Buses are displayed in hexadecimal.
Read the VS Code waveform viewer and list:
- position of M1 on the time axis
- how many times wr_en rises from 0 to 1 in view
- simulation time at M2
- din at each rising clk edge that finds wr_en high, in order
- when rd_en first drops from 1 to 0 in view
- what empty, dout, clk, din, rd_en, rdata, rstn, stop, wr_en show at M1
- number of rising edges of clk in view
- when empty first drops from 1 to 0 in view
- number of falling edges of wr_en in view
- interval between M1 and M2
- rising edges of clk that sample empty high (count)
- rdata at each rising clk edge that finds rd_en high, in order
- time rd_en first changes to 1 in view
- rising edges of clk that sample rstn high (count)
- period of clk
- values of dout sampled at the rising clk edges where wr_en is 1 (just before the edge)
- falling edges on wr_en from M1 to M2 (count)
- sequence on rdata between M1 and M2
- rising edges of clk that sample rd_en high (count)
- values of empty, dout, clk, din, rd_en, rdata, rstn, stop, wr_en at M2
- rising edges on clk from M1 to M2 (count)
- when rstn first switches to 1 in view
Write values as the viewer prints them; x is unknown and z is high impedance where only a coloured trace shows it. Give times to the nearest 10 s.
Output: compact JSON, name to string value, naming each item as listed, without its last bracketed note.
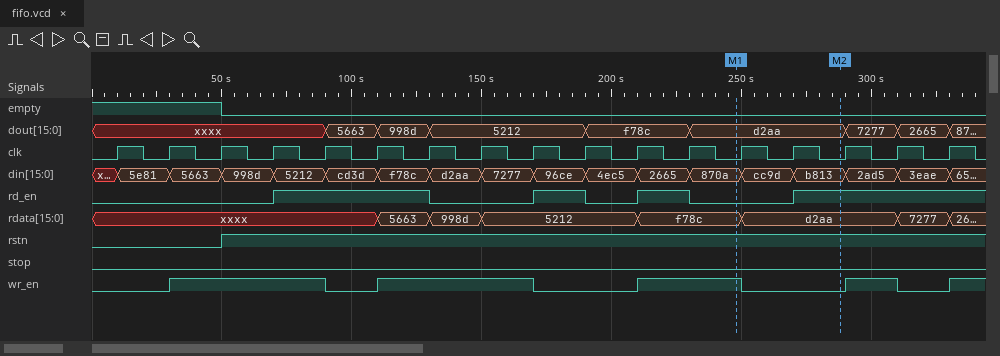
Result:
{"position of M1 on the time axis": "250 s", "how many times wr_en rises from 0 to 1 in view": "5", "simulation time at M2": "290 s", "din at each rising clk edge that finds wr_en high, in order": "5663, 998d, 5212, f78c, d2aa, 7277, 2665, 870a, 2ad5", "when rd_en first drops from 1 to 0 in view": "130 s", "what empty, dout, clk, din, rd_en, rdata, rstn, stop, wr_en show at M1": "empty=0, dout=d2aa, clk=0, din=870a, rd_en=0, rdata=f78c, rstn=1, stop=0, wr_en=1", "number of rising edges of clk in view": "17", "when empty first drops from 1 to 0 in view": "50 s", "number of falling edges of wr_en in view": "4", "interval between M1 and M2": "40 s", "rising edges of clk that sample empty high": "3", "rdata at each rising clk edge that finds rd_en high, in order": "xxxx, xxxx, 5663, 5212, f78c, d2aa, d2aa, 7277", "time rd_en first changes to 1 in view": "70 s", "rising edges of clk that sample rstn high": "14", "period of clk": "20 s", "values of dout sampled at the rising clk edges where wr_en is 1": "xxxx, xxxx, xxxx, 998d, 5212, 5212, f78c, d2aa, 7277", "falling edges on wr_en from M1 to M2": "1", "sequence on rdata between M1 and M2": "f78c, d2aa", "rising edges of clk that sample rd_en high": "8", "values of empty, dout, clk, din, rd_en, rdata, rstn, stop, wr_en at M2": "empty=0, dout=d2aa, clk=0, din=b813, rd_en=1, rdata=d2aa, rstn=1, stop=0, wr_en=0", "rising edges on clk from M1 to M2": "2", "when rstn first switches to 1 in view": "50 s"}
